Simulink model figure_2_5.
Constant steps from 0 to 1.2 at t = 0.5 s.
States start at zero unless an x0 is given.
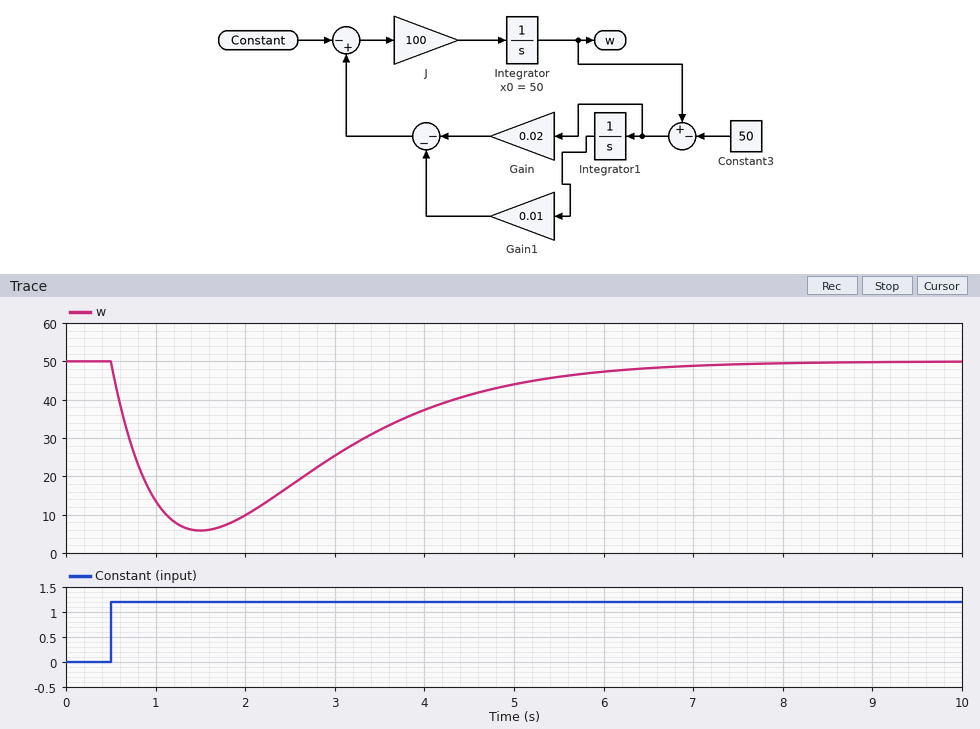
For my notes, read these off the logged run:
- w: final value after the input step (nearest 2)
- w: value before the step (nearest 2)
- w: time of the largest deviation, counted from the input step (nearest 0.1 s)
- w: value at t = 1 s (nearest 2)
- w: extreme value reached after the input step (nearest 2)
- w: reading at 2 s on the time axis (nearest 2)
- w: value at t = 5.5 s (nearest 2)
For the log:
50
50
1.0 s
14
6
10
46
